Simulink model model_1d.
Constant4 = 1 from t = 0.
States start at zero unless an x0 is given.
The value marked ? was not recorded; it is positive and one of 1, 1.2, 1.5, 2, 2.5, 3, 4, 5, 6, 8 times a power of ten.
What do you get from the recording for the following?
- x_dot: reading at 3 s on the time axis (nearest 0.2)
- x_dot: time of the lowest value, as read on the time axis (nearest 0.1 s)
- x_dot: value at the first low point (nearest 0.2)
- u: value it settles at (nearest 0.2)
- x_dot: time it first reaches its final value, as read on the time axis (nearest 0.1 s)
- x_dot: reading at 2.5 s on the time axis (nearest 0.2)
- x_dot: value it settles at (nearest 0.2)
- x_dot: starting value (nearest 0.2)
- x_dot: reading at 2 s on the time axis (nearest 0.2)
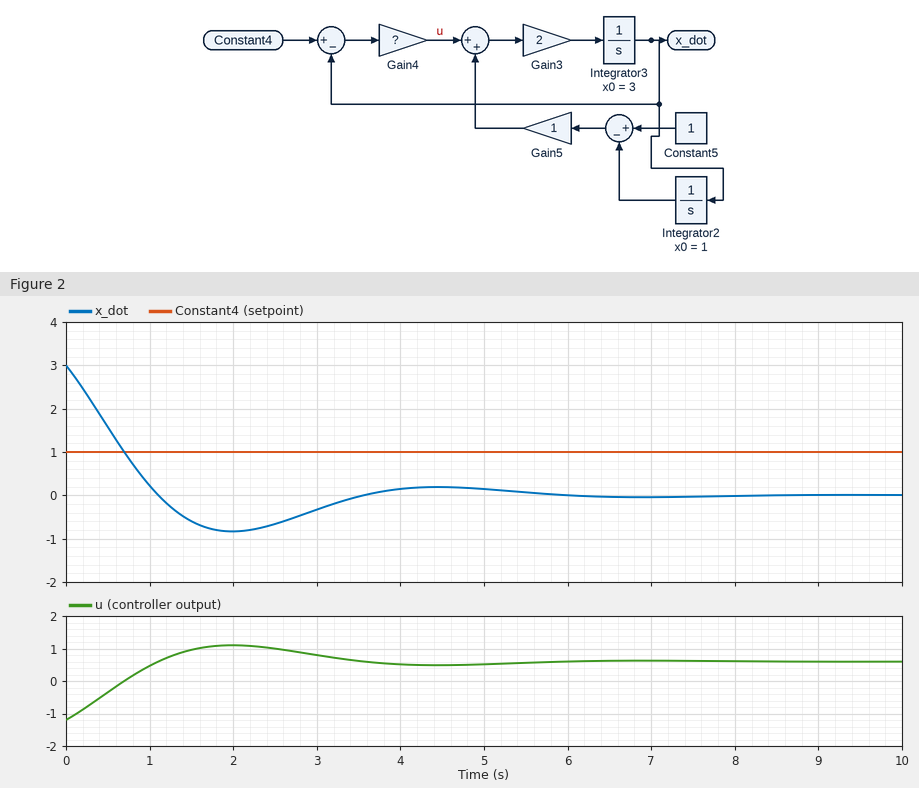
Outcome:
-0.4
2.0 s
-0.8
0.6
1.1 s
-0.6
0.0
3.0
-0.8
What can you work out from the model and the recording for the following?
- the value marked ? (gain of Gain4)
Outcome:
0.6
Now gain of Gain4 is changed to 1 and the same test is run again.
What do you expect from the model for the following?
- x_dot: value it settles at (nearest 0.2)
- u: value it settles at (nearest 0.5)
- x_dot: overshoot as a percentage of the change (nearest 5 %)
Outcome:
0.0
1.0
10 %
